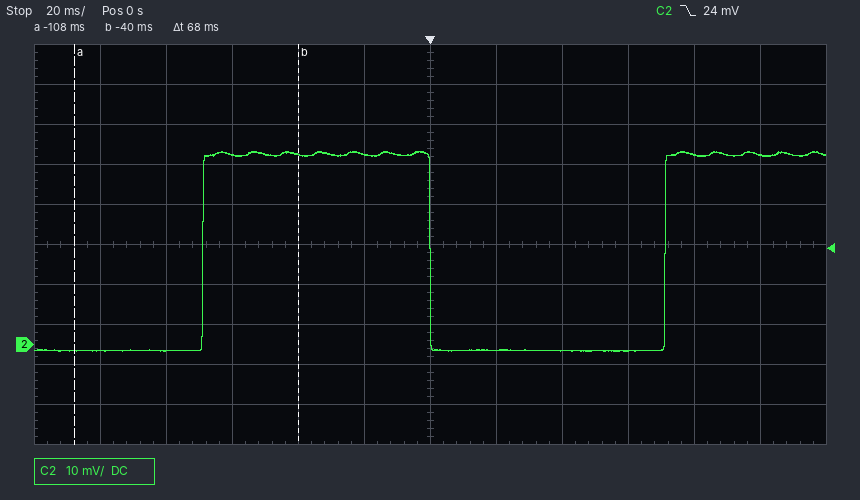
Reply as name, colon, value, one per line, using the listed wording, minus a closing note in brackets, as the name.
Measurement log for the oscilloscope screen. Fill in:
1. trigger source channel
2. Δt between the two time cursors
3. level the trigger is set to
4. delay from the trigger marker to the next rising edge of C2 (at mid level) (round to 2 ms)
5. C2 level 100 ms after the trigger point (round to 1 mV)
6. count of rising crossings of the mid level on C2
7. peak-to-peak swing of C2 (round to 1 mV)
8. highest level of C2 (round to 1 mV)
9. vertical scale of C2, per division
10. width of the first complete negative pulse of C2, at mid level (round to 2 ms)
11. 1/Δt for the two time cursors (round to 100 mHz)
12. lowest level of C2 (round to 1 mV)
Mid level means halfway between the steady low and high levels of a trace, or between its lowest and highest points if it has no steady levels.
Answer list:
trigger source channel: C2
Δt between the two time cursors: 68 ms
level the trigger is set to: 24 mV
delay from the trigger marker to the next rising edge of C2 (at mid level): 72 ms
C2 level 100 ms after the trigger point: 47 mV
count of rising crossings of the mid level on C2: 2
peak-to-peak swing of C2: 50 mV
highest level of C2: 48 mV
vertical scale of C2, per division: 10 mV
width of the first complete negative pulse of C2, at mid level: 72 ms
1/Δt for the two time cursors: 14.7 Hz
lowest level of C2: -2 mV
